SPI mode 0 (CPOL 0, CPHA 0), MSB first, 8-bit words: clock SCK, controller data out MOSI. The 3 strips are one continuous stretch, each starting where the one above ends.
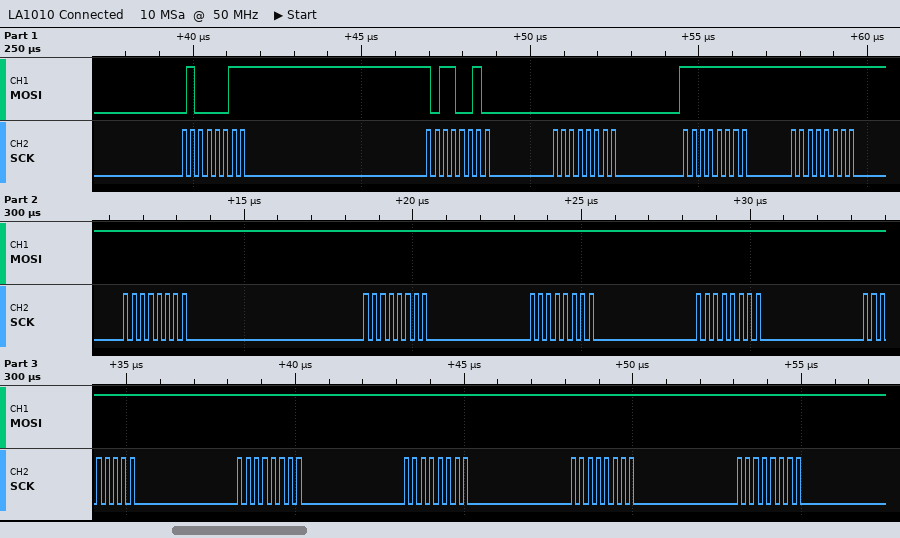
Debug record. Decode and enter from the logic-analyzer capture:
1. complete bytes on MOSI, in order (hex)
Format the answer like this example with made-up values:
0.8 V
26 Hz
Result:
43 B2 00 FF FF FF FF FF FF FF FF FF FF FF
